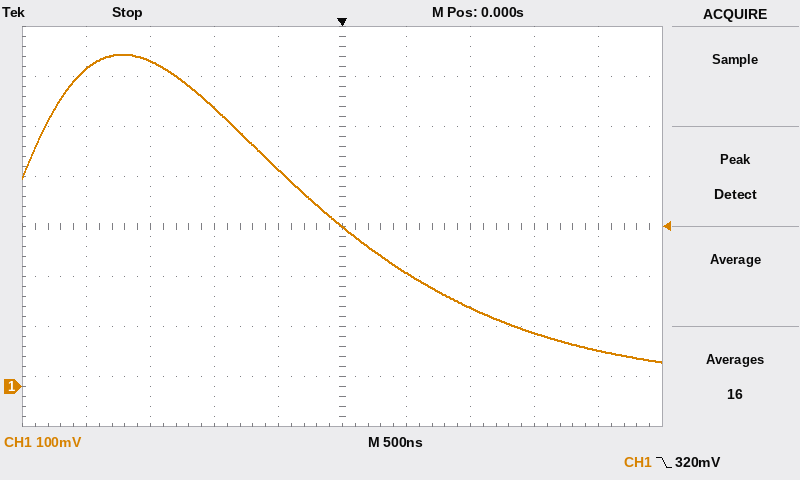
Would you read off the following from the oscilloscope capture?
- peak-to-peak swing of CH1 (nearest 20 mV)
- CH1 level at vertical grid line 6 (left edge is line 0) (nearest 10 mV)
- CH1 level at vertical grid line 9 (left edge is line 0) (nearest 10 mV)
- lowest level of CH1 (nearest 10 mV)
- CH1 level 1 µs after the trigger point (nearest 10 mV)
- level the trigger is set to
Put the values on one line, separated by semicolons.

620 mV; 230 mV; 70 mV; 50 mV; 160 mV; 320 mV
